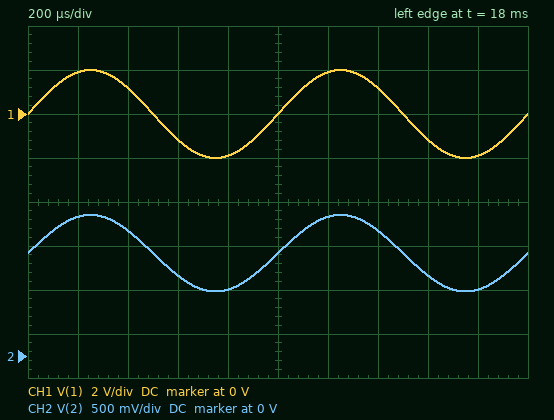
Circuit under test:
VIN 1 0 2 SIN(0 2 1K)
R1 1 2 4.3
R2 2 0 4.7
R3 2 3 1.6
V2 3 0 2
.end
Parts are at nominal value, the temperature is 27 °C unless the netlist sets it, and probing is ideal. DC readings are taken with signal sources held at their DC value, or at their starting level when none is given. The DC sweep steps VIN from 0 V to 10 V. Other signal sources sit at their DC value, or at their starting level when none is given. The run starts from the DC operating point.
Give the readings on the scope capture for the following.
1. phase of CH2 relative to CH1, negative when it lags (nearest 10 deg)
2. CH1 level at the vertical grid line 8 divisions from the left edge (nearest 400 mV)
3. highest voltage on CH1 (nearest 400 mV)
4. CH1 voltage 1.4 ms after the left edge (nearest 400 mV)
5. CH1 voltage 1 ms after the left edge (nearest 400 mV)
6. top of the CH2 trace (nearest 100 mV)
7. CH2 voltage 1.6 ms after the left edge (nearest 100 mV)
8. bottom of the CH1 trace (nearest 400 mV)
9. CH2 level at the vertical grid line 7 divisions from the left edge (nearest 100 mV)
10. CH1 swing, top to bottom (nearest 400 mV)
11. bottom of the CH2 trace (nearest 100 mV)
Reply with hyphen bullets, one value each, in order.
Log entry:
- 0 deg
- -1.2 V
- 2.0 V
- 1.2 V
- 0 V
- 1.6 V
- 900 mV
- -2.0 V
- 1.4 V
- 4.0 V
- 700 mV
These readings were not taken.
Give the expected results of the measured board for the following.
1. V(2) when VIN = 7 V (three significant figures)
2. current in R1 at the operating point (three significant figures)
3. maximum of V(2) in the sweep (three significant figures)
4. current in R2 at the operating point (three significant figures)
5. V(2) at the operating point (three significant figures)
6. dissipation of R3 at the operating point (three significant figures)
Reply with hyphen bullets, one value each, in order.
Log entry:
- 2.69 V
- 92.5 mA
- 3.34 V
- 341 mA
- 1.60 V
- 98.8 mW
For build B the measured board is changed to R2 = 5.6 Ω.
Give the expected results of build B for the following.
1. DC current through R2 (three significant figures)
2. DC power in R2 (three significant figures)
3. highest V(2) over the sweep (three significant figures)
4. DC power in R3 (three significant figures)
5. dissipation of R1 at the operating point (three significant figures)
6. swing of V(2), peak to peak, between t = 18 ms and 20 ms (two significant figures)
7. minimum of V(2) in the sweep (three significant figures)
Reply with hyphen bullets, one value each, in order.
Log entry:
- 296 mA
- 489 mW
- 3.45 V
- 74.3 mW
- 27.6 mW
- 900 mV
- 1.21 V
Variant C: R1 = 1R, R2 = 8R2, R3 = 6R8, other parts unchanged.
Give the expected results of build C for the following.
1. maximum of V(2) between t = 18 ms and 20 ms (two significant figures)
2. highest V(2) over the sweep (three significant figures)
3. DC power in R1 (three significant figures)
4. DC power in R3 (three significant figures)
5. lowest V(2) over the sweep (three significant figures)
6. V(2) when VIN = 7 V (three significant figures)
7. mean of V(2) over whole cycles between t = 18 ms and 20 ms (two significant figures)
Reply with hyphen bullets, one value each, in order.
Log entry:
- 1.8 V
- 8.11 V
- 36.9 mW
- 5.43 mW
- 232 mV
- 5.75 V
- 230 mV
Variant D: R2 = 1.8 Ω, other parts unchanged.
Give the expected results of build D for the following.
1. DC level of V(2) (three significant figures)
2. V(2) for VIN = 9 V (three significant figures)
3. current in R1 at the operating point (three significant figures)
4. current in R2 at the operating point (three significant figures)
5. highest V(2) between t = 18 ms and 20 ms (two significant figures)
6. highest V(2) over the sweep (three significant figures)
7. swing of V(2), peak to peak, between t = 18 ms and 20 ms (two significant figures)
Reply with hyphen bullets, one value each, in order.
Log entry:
- 1.21 V
- 2.37 V
- 183 mA
- 674 mA
- 1.2 V
- 2.53 V
- 660 mV
